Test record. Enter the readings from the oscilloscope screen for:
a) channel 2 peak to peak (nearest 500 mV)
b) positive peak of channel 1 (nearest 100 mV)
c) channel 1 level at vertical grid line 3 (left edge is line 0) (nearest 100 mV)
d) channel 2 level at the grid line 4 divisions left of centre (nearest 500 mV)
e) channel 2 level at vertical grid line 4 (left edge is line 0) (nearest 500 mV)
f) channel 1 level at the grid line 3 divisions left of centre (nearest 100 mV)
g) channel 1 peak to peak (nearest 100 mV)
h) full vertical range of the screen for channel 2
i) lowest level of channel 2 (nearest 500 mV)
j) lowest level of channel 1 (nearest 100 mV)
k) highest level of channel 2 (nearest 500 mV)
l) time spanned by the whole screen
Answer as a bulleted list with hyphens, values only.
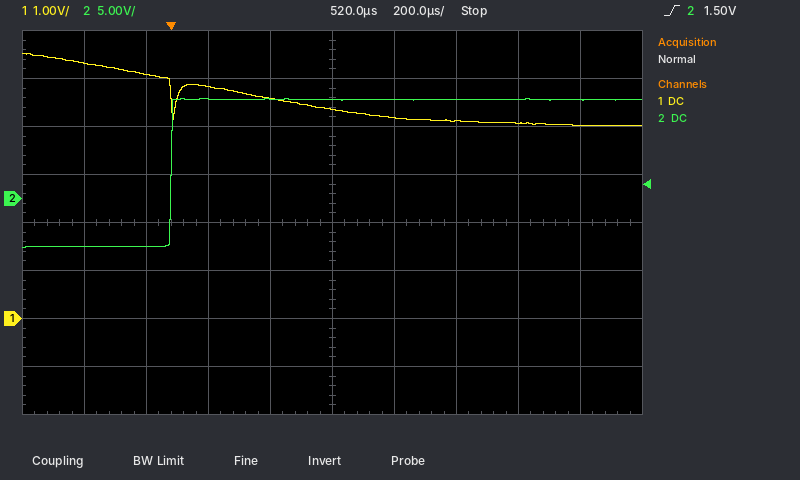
- 15.5 V
- 5.5 V
- 4.8 V
- -5.0 V
- 10.5 V
- 5.1 V
- 1.5 V
- 40 V
- -5.0 V
- 4.0 V
- 10.5 V
- 2 ms
